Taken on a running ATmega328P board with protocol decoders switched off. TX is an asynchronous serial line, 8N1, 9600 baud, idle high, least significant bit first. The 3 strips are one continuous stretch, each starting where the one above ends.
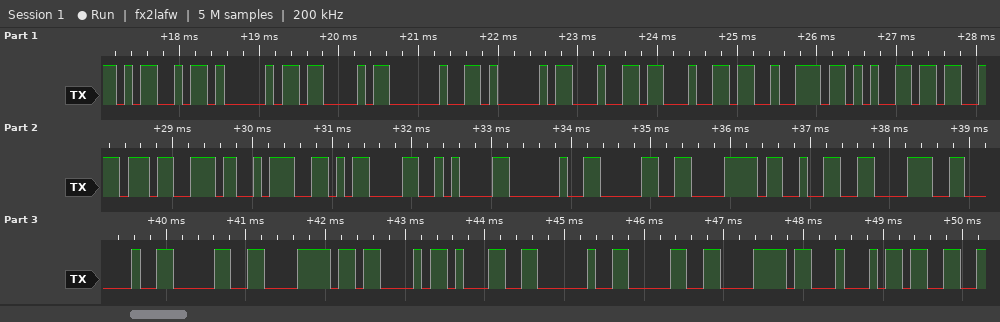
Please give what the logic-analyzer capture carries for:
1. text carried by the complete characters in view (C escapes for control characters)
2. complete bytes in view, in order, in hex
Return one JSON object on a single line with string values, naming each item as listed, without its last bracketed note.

{"text carried by the complete characters in view": "\"MAC Address:\\r\\n 0x28 0xC1 0xD3\"", "complete bytes in view, in order, in hex": "4D 41 43 20 41 64 64 72 65 73 73 3A 0D 0A 20 30 78 32 38 20 30 78 43 31 20 30 78 44 33"}
